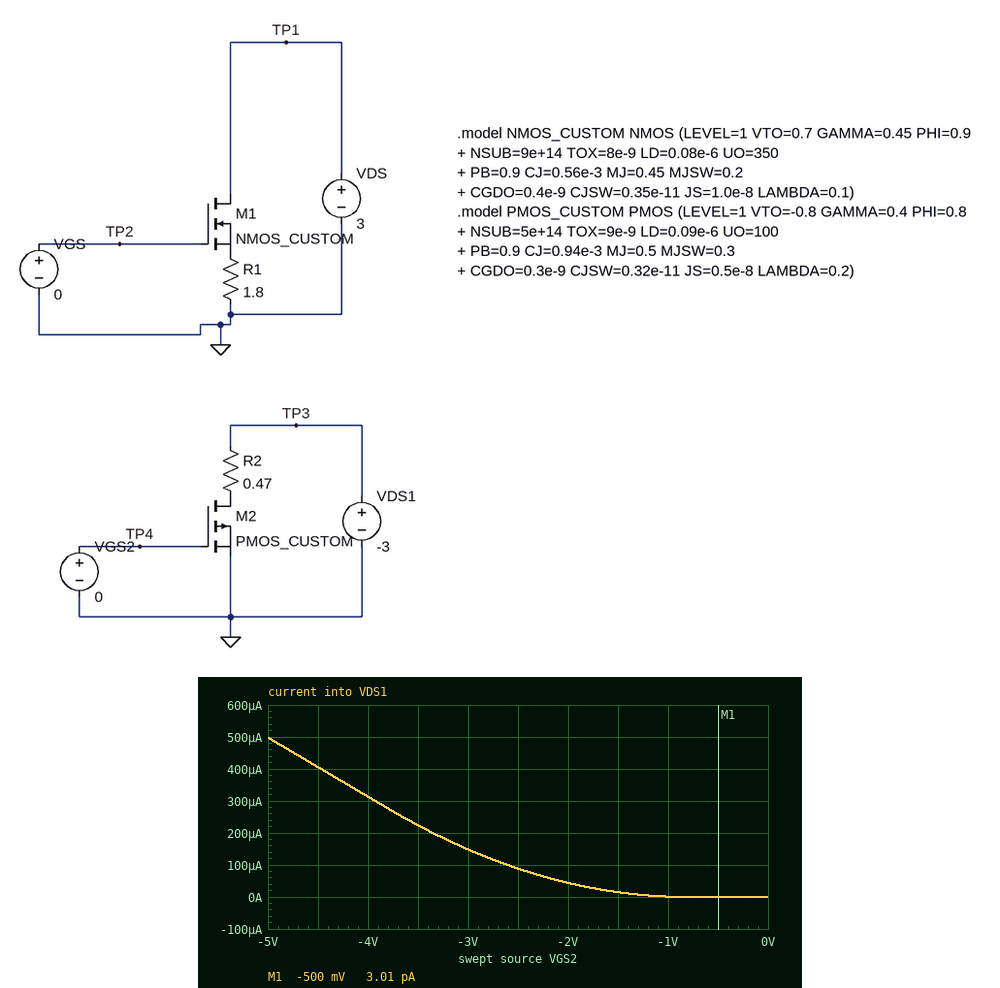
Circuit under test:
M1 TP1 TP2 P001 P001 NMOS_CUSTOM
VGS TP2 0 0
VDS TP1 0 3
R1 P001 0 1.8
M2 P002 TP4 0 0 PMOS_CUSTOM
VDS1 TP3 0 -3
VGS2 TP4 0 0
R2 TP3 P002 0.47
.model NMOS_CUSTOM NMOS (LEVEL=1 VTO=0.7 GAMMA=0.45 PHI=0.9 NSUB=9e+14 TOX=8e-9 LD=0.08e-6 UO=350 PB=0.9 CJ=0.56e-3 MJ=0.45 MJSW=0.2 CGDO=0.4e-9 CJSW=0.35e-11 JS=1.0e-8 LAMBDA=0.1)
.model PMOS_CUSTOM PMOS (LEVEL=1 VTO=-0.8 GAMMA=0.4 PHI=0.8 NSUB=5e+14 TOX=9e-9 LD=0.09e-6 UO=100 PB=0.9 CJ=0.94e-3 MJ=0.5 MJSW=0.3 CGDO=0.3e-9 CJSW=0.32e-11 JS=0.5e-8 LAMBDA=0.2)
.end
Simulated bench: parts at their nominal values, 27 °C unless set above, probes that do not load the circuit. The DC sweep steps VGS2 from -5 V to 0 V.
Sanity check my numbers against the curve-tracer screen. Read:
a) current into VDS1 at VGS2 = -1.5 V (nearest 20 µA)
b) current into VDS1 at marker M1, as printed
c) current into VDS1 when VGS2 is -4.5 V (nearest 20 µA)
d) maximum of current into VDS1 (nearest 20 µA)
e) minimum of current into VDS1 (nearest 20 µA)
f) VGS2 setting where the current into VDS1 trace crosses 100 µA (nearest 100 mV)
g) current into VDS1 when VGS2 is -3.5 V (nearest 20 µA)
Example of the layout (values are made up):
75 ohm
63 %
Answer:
20 µA
3.01 pA
400 µA
500 µA
0 A
-2.6 V
220 µA
